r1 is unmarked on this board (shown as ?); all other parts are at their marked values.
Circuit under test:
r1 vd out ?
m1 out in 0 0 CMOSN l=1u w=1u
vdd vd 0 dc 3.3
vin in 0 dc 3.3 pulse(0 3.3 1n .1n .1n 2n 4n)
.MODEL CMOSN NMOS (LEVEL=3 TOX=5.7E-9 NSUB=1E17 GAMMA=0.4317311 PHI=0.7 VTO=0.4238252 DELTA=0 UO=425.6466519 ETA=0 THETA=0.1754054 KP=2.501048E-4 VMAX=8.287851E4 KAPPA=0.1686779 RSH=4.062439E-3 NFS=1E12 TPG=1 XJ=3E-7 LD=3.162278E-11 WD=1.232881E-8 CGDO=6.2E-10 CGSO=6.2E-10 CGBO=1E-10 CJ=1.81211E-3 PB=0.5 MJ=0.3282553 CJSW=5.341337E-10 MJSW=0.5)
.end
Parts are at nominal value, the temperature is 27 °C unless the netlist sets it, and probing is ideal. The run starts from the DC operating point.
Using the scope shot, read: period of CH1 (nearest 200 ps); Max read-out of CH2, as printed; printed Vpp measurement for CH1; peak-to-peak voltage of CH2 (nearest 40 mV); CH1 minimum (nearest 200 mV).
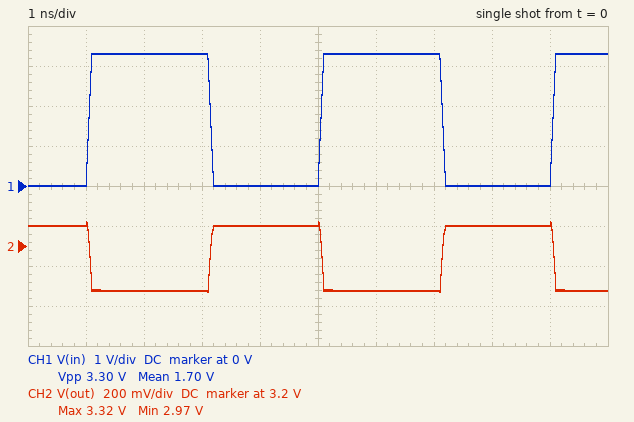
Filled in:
4.0 ns
3.32 V
3.30 V
360 mV
0 V
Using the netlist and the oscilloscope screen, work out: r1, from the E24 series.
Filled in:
910 Ω
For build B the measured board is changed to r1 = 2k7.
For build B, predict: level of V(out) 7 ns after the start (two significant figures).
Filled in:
2.4 V
